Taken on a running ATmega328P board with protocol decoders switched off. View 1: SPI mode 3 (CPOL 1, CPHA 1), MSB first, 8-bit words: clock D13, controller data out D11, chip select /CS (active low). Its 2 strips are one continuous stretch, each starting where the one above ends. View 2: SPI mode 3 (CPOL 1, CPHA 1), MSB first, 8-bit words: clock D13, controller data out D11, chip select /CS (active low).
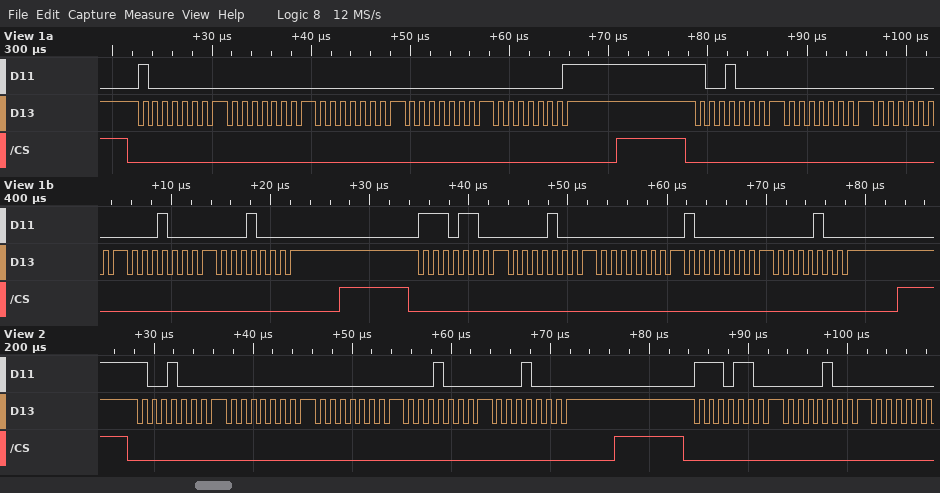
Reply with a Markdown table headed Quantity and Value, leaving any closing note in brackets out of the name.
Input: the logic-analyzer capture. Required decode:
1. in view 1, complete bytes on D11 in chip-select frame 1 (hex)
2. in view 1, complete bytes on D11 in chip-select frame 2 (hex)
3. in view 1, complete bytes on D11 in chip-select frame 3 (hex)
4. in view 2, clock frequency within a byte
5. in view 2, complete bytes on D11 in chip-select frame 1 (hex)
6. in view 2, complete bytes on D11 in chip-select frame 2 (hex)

| Quantity | Value |
|---|---|
| in view 1, complete bytes on D11 in chip-select frame 1 | 0x80 0x00 0x00 0x00 0x01 |
| in view 1, complete bytes on D11 in chip-select frame 2 | 0x90 0x00 0x00 0x10 0x10 |
| in view 1, complete bytes on D11 in chip-select frame 3 | 0xEC 0x08 0x00 0x80 0x08 |
| in view 2, clock frequency within a byte | 1 MHz |
| in view 2, complete bytes on D11 in chip-select frame 1 | 90 00 00 10 10 |
| in view 2, complete bytes on D11 in chip-select frame 2 | EC 08 |
